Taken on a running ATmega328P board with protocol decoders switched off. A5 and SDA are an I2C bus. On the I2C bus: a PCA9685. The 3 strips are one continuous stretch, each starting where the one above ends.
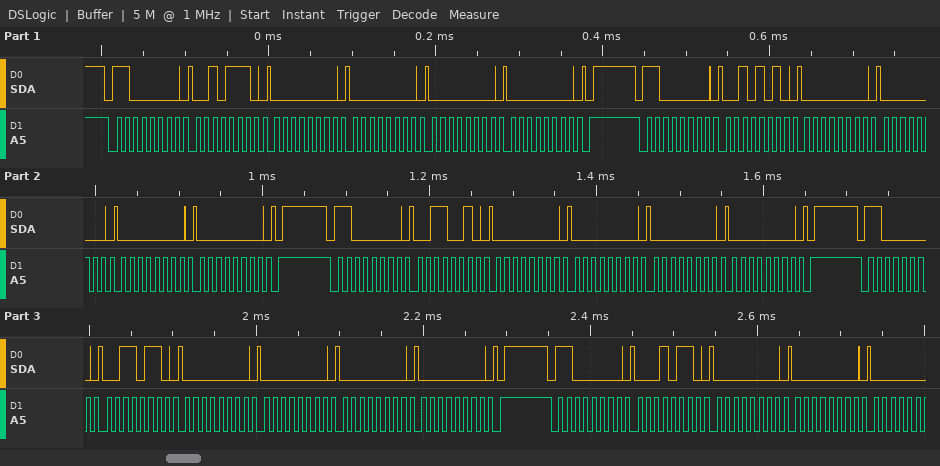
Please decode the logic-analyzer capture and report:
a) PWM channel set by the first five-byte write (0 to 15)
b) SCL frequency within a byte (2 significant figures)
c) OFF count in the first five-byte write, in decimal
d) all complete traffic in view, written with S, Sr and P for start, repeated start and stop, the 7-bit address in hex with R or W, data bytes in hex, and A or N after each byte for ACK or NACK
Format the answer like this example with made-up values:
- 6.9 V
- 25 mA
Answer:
- 10
- 100 kHz
- 0
- S 60W A 2E A 00 A 00 A 00 A 00 A P S 60W A 2A A 00 A 00 A 00 A 00 A P S 60W A 32 A 00 A 00 A 00 A 00 A P S 60W A 36 A 00 A 00 A 00 A 00 A P S 60W A 16 A 00 A 00 A
